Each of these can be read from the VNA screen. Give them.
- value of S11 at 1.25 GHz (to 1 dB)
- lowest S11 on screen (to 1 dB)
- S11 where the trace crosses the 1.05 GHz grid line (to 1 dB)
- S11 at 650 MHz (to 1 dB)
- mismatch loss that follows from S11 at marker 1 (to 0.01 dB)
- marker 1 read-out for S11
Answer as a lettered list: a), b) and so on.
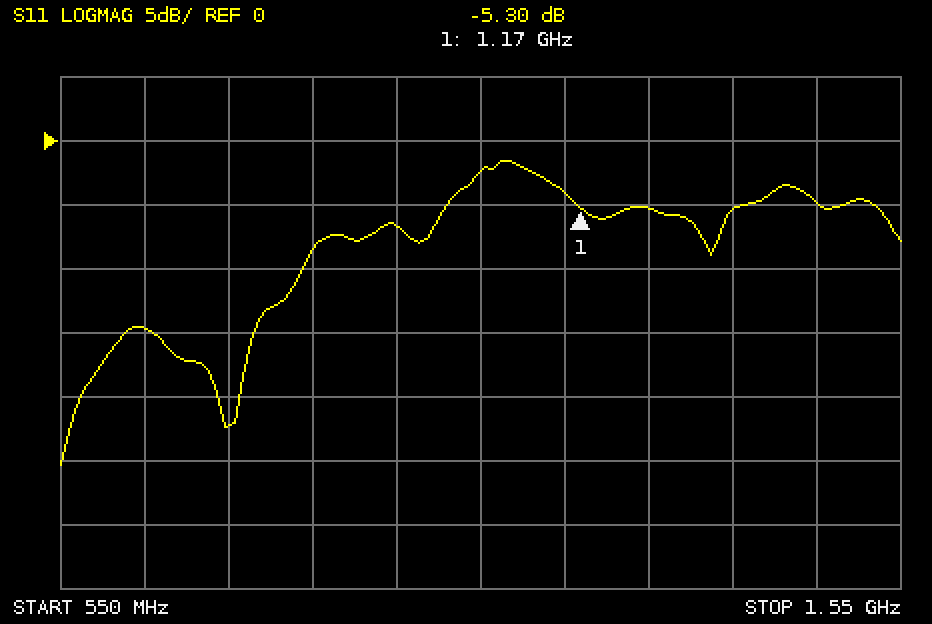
a) -5 dB
b) -25 dB
c) -2 dB
d) -15 dB
e) 1.52 dB
f) -5.30 dB
